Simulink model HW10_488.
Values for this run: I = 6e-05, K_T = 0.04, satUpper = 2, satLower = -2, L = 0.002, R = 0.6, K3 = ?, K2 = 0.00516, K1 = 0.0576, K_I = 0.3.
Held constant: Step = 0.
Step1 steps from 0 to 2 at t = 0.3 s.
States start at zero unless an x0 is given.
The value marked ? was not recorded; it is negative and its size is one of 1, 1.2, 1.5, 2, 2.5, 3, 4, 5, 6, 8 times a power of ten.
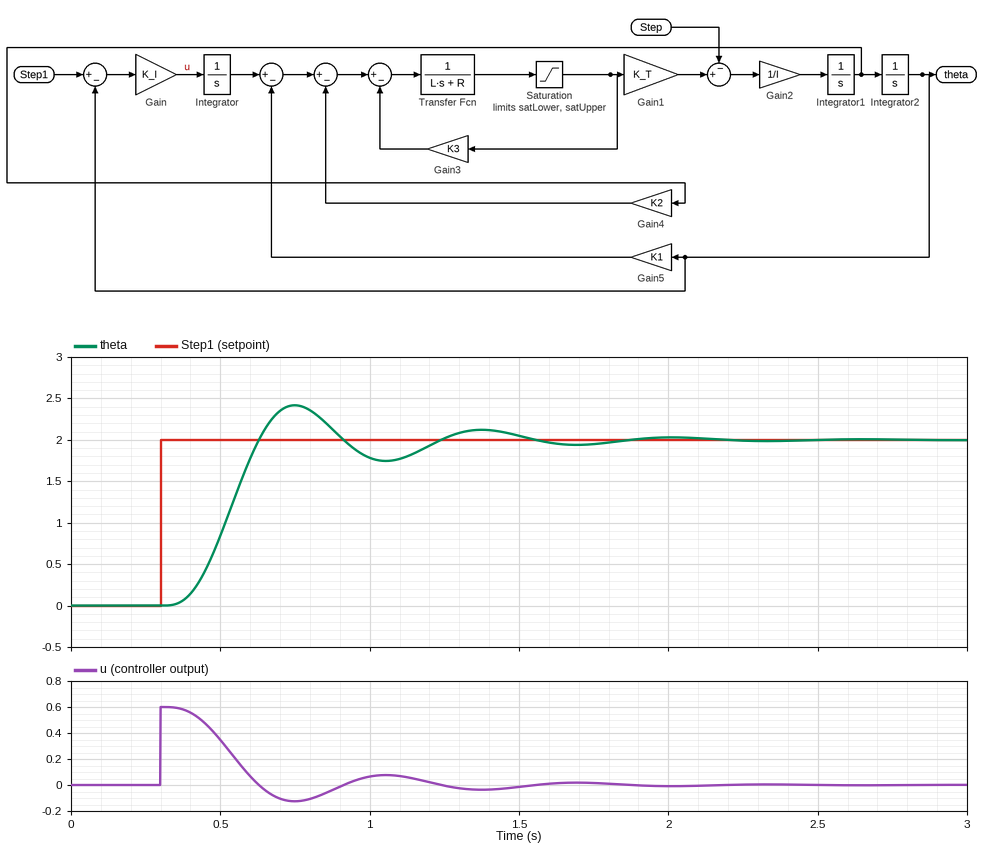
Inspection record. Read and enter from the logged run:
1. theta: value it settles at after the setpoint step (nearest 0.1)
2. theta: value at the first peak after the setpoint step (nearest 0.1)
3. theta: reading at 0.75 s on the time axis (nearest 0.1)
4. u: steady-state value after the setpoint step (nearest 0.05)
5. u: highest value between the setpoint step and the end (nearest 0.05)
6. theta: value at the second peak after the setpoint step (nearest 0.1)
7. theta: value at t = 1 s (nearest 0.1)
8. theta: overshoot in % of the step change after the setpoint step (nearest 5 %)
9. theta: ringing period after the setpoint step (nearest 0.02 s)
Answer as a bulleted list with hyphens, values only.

- 2.0
- 2.4
- 2.4
- 0.00
- 0.60
- 2.1
- 1.8
- 20 %
- 0.62 s
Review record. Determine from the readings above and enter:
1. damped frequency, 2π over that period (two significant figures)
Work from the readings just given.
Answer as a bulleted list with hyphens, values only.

- 10 rad/s
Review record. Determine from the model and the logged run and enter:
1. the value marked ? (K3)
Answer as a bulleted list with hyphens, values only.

- -0.3
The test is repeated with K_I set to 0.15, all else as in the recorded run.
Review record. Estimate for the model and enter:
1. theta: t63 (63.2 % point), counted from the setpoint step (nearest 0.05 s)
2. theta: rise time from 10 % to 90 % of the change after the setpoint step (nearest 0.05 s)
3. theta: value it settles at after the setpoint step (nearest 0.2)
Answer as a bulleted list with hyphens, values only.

- 0.35 s
- 0.65 s
- 2.0
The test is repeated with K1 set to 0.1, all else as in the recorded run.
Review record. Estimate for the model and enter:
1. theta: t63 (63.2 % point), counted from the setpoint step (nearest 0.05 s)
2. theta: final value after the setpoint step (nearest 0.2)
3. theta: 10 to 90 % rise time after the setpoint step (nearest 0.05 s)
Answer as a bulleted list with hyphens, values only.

- 0.30 s
- 2.0
- 0.60 s
